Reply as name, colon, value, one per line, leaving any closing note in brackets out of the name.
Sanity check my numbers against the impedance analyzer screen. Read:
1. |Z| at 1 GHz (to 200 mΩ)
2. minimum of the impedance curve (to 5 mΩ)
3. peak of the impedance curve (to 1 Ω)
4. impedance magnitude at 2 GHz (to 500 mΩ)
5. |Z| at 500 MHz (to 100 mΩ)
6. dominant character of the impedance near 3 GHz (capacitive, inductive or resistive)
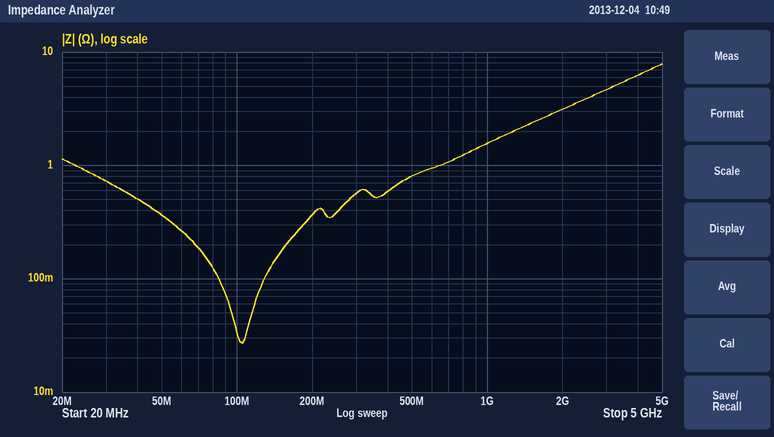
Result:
|Z| at 1 GHz: 1.6 Ω
minimum of the impedance curve: 25 mΩ
peak of the impedance curve: 8 Ω
impedance magnitude at 2 GHz: 3.0 Ω
|Z| at 500 MHz: 800 mΩ
dominant character of the impedance near 3 GHz: inductive
